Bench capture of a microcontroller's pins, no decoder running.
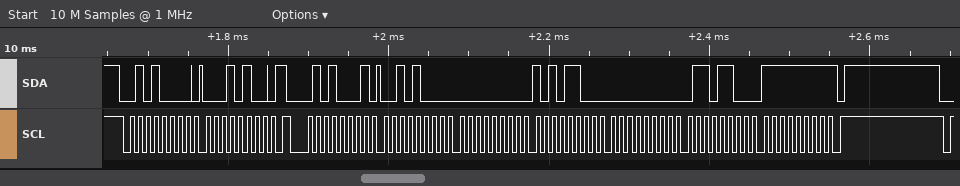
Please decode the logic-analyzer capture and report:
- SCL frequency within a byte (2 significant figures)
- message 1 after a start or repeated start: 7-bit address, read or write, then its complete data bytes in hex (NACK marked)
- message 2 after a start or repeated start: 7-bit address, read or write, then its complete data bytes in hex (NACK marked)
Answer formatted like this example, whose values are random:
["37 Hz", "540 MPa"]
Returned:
["100 kHz", "0x28 write: 14", "0x28 read: 28 00 AC 00 6C FF NACK"]
